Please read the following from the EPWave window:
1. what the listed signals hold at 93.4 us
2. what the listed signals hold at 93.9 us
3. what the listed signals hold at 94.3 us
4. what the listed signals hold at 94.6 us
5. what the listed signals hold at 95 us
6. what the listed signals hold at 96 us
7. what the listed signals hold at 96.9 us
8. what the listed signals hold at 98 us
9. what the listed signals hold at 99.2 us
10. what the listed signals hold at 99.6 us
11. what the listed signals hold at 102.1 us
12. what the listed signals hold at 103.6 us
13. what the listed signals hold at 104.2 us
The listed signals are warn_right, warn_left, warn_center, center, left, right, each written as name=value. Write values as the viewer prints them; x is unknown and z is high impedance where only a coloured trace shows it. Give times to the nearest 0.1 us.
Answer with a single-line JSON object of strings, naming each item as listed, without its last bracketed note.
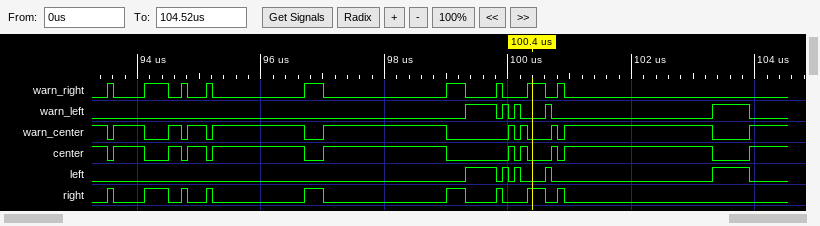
{"what the listed signals hold at 93.4 us": "warn_right=0, warn_left=0, warn_center=1, center=1, left=0, right=0", "what the listed signals hold at 93.9 us": "warn_right=0, warn_left=0, warn_center=1, center=1, left=0, right=0", "what the listed signals hold at 94.3 us": "warn_right=1, warn_left=0, warn_center=0, center=0, left=0, right=1", "what the listed signals hold at 94.6 us": "warn_right=0, warn_left=0, warn_center=1, center=1, left=0, right=0", "what the listed signals hold at 95 us": "warn_right=0, warn_left=0, warn_center=1, center=1, left=0, right=0", "what the listed signals hold at 96 us": "warn_right=0, warn_left=0, warn_center=1, center=1, left=0, right=0", "what the listed signals hold at 96.9 us": "warn_right=1, warn_left=0, warn_center=0, center=0, left=0, right=1", "what the listed signals hold at 98 us": "warn_right=0, warn_left=0, warn_center=1, center=1, left=0, right=0", "what the listed signals hold at 99.2 us": "warn_right=1, warn_left=0, warn_center=0, center=0, left=0, right=1", "what the listed signals hold at 99.6 us": "warn_right=0, warn_left=1, warn_center=0, center=0, left=1, right=0", "what the listed signals hold at 102.1 us": "warn_right=0, warn_left=0, warn_center=1, center=1, left=0, right=0", "what the listed signals hold at 103.6 us": "warn_right=0, warn_left=1, warn_center=0, center=0, left=1, right=0", "what the listed signals hold at 104.2 us": "warn_right=0, warn_left=0, warn_center=1, center=1, left=0, right=0"}
